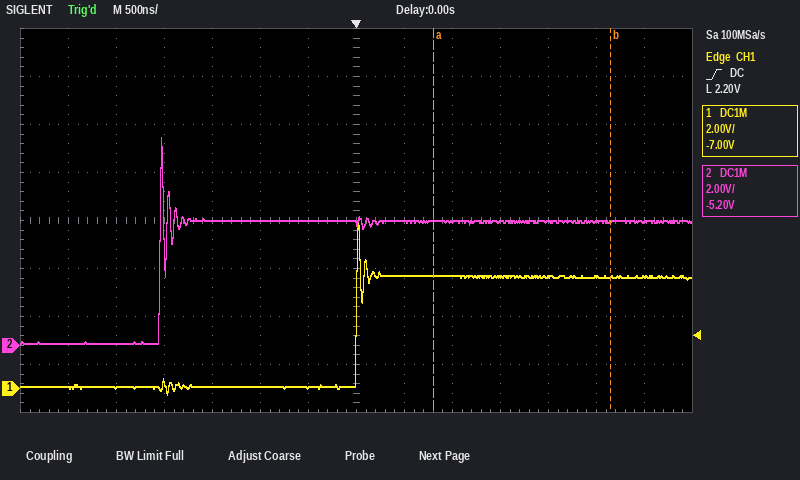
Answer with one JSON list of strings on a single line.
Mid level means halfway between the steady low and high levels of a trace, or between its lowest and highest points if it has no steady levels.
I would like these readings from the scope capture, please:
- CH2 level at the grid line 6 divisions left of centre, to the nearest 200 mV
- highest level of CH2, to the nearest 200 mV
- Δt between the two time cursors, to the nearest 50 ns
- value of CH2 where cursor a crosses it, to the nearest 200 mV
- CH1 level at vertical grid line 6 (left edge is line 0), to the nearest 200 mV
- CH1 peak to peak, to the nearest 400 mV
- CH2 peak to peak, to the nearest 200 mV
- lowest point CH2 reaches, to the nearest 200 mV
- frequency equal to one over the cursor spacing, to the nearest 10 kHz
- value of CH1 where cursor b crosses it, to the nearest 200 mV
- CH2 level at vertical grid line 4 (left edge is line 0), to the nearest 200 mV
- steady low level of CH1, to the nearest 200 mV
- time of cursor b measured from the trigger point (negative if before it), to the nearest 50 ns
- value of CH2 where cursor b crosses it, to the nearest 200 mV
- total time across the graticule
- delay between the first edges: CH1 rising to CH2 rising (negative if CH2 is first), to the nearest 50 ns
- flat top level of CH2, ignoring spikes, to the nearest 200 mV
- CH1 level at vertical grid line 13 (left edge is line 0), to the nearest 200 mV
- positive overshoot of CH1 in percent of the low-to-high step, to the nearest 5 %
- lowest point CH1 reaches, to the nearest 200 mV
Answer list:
["0.0 V", "8.6 V", "1.85 µs", "5.2 V", "0.0 V", "7.2 V", "8.6 V", "0.0 V", "540 kHz", "4.6 V", "5.2 V", "0.0 V", "+2.65 µs", "5.2 V", "7 µs", "-2.05 µs", "5.2 V", "4.6 V", "50 %", "-200 mV"]
